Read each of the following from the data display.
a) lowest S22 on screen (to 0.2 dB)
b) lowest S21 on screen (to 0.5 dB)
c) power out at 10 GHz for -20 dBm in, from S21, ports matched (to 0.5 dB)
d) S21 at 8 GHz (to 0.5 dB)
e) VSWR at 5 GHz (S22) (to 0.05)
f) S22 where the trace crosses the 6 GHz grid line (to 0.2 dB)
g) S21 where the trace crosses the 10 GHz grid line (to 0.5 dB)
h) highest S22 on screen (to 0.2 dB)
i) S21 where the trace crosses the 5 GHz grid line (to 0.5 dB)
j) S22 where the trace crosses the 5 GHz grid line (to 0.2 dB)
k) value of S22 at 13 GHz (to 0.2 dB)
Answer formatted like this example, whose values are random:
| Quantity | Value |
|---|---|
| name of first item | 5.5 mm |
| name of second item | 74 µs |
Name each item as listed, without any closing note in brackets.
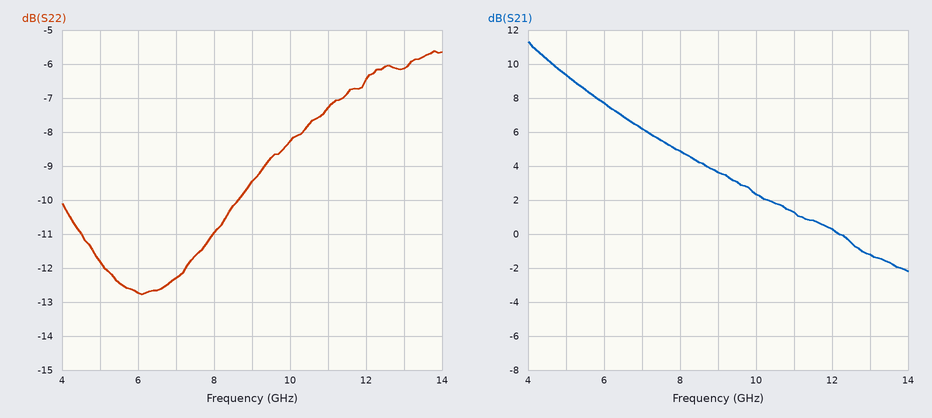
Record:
| Quantity | Value |
|---|---|
| lowest S22 on screen | -12.8 dB |
| lowest S21 on screen | -2.0 dB |
| power out at 10 GHz for -20 dBm in, from S21, ports matched | -17.5 dBm |
| S21 at 8 GHz | 5.0 dB |
| VSWR at 5 GHz (S22) | 1.70 |
| S22 where the trace crosses the 6 GHz grid line | -12.8 dB |
| S21 where the trace crosses the 10 GHz grid line | 2.5 dB |
| highest S22 on screen | -5.6 dB |
| S21 where the trace crosses the 5 GHz grid line | 9.5 dB |
| S22 where the trace crosses the 5 GHz grid line | -11.8 dB |
| value of S22 at 13 GHz | -6.2 dB |
